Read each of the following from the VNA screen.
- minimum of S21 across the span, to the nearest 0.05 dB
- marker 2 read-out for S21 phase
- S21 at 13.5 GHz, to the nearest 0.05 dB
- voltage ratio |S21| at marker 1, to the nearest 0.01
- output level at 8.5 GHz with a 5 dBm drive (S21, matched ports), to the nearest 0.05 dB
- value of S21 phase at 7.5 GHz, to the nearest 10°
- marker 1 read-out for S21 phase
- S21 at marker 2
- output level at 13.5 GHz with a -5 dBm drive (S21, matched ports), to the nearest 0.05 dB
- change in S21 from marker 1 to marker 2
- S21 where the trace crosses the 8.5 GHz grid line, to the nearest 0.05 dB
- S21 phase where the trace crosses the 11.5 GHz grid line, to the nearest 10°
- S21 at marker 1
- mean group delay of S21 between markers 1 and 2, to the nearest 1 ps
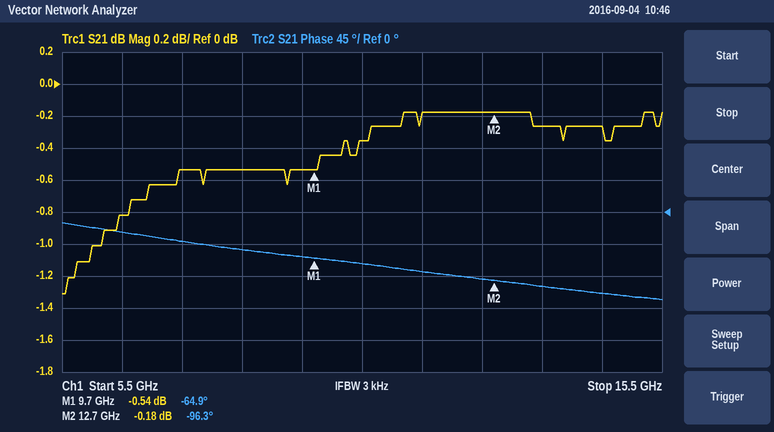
-1.30 dB
-96.3°
-0.25 dB
0.94
4.45 dBm
-40°
-64.9°
-0.18 dB
-5.25 dBm
0.36 dB
-0.55 dB
-80°
-0.54 dB
29 ps
